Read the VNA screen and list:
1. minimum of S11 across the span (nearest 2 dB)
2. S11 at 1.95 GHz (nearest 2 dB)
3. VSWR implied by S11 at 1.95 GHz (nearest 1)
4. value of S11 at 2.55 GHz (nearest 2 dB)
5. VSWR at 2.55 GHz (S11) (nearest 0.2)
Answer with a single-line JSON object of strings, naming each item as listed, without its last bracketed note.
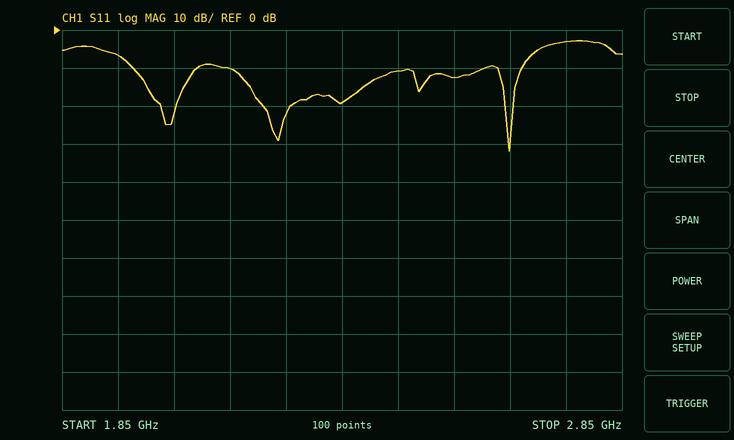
{"minimum of S11 across the span": "-32 dB", "S11 at 1.95 GHz": "-6 dB", "VSWR implied by S11 at 1.95 GHz": "3", "value of S11 at 2.55 GHz": "-12 dB", "VSWR at 2.55 GHz (S11)": "1.6"}
